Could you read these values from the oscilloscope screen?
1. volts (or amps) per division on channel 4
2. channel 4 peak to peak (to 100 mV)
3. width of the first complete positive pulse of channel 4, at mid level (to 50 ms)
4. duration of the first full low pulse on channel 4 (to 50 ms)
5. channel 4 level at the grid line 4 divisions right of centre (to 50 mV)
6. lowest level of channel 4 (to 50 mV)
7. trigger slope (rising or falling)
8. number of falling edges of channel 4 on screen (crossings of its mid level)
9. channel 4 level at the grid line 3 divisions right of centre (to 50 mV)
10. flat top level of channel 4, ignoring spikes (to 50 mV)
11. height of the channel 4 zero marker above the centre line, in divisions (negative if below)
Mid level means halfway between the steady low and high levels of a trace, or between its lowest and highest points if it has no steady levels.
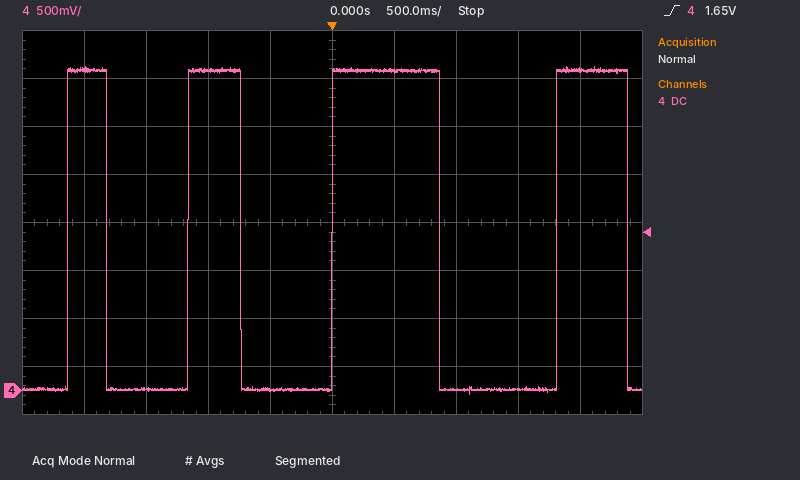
500 mV
3.40 V
300 ms
650 ms
3.35 V
-50 mV
rising
4
0 mV
3.35 V
-3.5 div
